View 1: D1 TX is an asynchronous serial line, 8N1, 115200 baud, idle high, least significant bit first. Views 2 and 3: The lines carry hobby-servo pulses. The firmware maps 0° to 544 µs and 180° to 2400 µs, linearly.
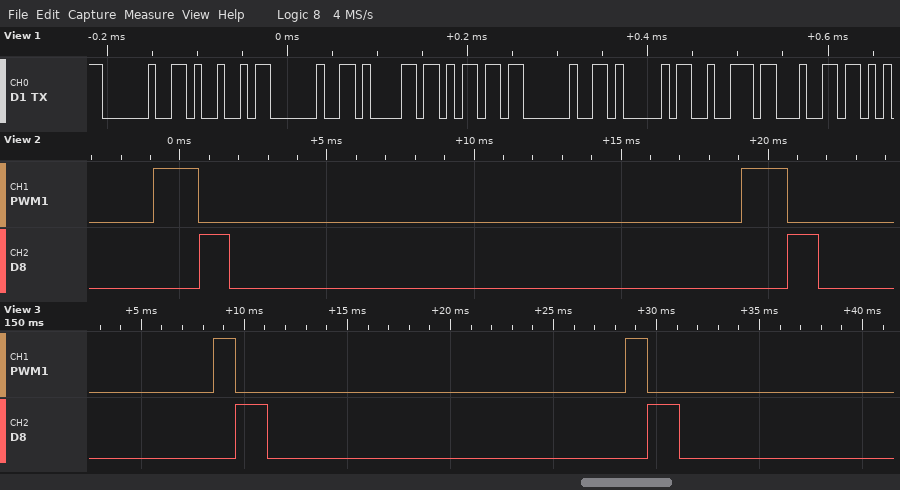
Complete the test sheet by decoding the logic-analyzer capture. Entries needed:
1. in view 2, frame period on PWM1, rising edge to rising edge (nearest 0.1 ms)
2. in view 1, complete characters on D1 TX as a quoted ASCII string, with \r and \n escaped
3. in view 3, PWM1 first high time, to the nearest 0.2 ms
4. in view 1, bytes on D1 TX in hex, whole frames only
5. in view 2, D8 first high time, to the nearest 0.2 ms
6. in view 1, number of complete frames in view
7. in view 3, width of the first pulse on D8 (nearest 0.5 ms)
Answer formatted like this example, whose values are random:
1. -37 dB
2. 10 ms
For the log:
1. 20.0 ms
2. " I am Ard"
3. 1.0 ms
4. 20 49 20 61 6D 20 41 72 64
5. 1.0 ms
6. 9
7. 1.5 ms
